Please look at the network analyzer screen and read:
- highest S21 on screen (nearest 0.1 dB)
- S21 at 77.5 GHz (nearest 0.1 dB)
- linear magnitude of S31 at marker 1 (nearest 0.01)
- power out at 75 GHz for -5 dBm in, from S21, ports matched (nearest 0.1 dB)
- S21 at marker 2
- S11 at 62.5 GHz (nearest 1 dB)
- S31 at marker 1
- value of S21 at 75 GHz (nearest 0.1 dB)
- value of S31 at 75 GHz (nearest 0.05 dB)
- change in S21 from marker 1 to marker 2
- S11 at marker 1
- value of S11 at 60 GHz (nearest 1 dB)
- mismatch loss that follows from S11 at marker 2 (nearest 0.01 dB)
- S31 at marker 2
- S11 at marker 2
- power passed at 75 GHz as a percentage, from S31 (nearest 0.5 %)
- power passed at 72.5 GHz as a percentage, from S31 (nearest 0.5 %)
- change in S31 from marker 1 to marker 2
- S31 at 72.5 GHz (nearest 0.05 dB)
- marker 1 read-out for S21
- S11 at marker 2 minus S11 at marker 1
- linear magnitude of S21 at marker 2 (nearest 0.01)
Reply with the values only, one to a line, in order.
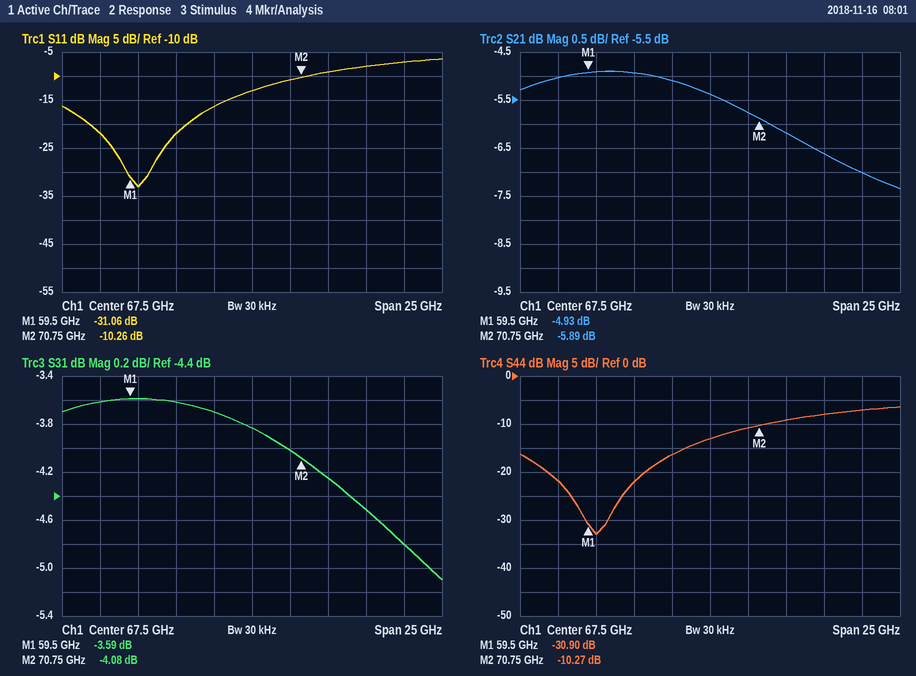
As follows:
-4.9 dB
-7.0 dB
0.66
-11.6 dBm
-5.89 dB
-22 dB
-3.59 dB
-6.6 dB
-4.50 dB
-0.96 dB
-31.06 dB
-33 dB
0.43 dB
-4.08 dB
-10.26 dB
35.5 %
37.5 %
-0.49 dB
-4.25 dB
-4.93 dB
20.80 dB
0.51
